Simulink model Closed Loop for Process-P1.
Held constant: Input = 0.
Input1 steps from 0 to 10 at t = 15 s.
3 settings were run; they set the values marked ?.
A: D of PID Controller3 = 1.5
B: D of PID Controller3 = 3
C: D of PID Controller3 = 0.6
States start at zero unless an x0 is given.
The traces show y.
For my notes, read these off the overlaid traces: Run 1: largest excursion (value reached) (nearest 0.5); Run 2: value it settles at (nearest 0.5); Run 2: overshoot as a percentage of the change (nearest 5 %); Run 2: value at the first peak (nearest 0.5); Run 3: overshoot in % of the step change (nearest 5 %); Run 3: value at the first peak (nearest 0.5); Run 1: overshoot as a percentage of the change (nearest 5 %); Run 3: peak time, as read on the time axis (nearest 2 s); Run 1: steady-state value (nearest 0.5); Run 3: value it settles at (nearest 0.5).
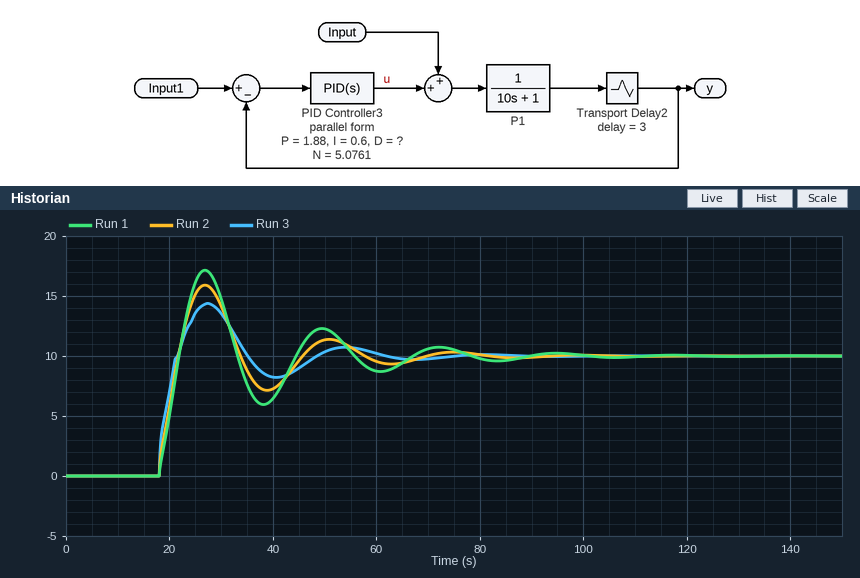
17.0
10.0
60 %
16.0
45 %
14.5
70 %
28 s
10.0
10.0
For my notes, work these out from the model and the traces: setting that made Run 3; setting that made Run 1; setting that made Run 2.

B
C
A
